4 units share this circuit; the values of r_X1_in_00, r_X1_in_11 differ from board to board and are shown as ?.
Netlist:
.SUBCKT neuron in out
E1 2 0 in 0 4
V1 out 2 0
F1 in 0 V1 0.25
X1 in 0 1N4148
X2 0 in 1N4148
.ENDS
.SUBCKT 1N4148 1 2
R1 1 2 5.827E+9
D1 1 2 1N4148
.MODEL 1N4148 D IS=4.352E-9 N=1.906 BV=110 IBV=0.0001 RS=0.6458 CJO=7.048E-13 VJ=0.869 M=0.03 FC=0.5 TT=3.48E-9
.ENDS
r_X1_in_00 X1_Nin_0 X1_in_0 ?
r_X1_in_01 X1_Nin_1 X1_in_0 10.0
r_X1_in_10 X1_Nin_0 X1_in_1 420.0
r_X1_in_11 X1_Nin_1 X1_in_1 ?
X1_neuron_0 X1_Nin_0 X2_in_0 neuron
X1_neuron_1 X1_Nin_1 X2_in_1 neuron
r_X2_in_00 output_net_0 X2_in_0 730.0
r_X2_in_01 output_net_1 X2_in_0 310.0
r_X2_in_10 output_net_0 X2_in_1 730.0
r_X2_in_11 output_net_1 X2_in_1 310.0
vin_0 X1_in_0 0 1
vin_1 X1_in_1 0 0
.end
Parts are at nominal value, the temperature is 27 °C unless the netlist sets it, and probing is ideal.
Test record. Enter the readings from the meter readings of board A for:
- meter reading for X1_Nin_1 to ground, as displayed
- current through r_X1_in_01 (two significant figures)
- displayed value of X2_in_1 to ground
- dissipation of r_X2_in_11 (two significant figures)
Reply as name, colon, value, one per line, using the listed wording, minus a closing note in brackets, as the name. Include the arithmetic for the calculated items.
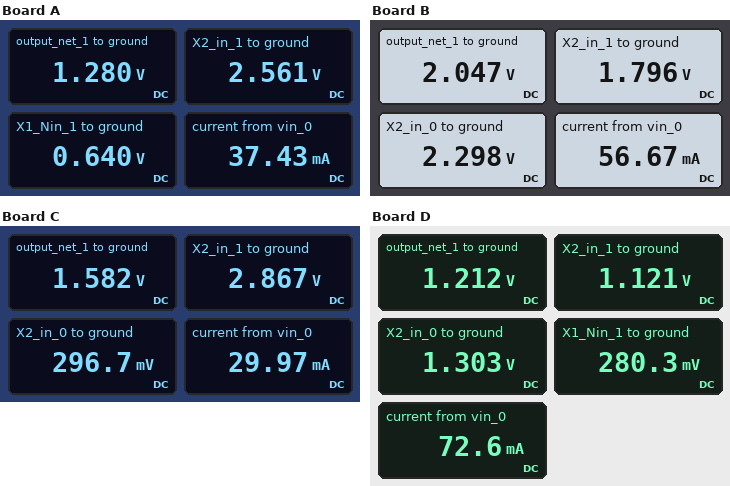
meter reading for X1_Nin_1 to ground, as displayed: 0.640 V
current through r_X1_in_01: (1 V - 640 mV) / 10 Ω = 36 mA
displayed value of X2_in_1 to ground: 2.561 V
dissipation of r_X2_in_11: (2.561 V - 1.28 V)^2 / 310 Ω = 5.3 mW
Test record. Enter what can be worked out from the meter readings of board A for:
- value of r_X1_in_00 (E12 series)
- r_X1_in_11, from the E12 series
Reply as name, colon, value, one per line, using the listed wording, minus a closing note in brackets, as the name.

value of r_X1_in_00: 680 Ω
r_X1_in_11, from the E12 series: 18 Ω
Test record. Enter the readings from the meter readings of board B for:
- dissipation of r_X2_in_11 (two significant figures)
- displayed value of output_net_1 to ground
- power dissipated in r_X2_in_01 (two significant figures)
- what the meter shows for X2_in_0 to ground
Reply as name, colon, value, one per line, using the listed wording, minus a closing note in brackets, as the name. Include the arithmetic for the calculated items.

dissipation of r_X2_in_11: (2.047 V - 1.796 V)^2 / 310 Ω = 200 µW
displayed value of output_net_1 to ground: 2.047 V
power dissipated in r_X2_in_01: (2.298 V - 2.047 V)^2 / 310 Ω = 200 µW
what the meter shows for X2_in_0 to ground: 2.298 V
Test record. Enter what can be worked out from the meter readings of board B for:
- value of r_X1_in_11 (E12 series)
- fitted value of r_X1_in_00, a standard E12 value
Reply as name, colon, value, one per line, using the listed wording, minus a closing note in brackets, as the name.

value of r_X1_in_11: 8.2 Ω
fitted value of r_X1_in_00, a standard E12 value: 270 Ω
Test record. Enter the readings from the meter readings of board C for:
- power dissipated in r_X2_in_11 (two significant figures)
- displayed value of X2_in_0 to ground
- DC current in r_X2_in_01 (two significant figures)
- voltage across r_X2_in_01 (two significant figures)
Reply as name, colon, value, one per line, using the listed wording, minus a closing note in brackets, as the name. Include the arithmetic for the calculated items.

power dissipated in r_X2_in_11: (2.867 V - 1.582 V)^2 / 310 Ω = 5.3 mW
displayed value of X2_in_0 to ground: 296.7 mV
DC current in r_X2_in_01: (1.582 V - 296.7 mV) / 310 Ω = 4.1 mA
voltage across r_X2_in_01: 1.582 V - 296.7 mV = 1.3 V
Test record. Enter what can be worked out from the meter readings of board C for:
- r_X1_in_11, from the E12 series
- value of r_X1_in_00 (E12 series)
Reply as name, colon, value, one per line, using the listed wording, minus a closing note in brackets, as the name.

r_X1_in_11, from the E12 series: 33 Ω
value of r_X1_in_00: 560 Ω
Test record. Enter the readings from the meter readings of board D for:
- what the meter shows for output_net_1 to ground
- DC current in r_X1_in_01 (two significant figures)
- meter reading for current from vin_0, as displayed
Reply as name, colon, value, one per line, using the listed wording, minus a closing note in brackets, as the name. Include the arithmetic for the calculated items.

what the meter shows for output_net_1 to ground: 1.212 V
DC current in r_X1_in_01: (1 V - 280.3 mV) / 10 Ω = 72 mA
meter reading for current from vin_0, as displayed: 72.6 mA
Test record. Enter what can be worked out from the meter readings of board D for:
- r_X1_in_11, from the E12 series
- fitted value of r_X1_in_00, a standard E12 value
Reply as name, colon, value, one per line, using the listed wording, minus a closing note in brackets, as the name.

r_X1_in_11, from the E12 series: 3.9 Ω
fitted value of r_X1_in_00, a standard E12 value: 1 kΩ
